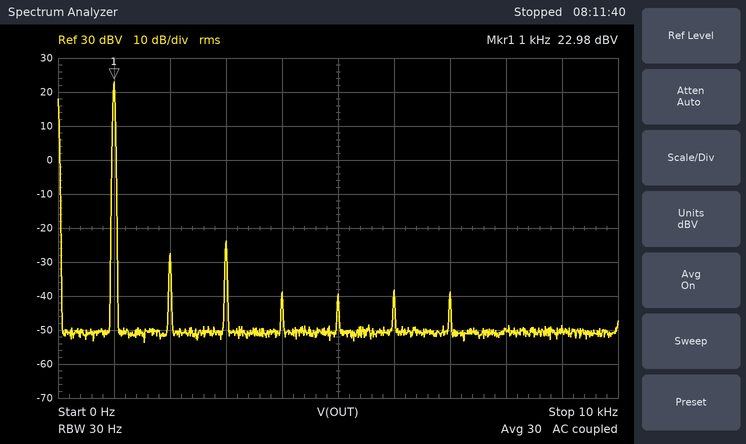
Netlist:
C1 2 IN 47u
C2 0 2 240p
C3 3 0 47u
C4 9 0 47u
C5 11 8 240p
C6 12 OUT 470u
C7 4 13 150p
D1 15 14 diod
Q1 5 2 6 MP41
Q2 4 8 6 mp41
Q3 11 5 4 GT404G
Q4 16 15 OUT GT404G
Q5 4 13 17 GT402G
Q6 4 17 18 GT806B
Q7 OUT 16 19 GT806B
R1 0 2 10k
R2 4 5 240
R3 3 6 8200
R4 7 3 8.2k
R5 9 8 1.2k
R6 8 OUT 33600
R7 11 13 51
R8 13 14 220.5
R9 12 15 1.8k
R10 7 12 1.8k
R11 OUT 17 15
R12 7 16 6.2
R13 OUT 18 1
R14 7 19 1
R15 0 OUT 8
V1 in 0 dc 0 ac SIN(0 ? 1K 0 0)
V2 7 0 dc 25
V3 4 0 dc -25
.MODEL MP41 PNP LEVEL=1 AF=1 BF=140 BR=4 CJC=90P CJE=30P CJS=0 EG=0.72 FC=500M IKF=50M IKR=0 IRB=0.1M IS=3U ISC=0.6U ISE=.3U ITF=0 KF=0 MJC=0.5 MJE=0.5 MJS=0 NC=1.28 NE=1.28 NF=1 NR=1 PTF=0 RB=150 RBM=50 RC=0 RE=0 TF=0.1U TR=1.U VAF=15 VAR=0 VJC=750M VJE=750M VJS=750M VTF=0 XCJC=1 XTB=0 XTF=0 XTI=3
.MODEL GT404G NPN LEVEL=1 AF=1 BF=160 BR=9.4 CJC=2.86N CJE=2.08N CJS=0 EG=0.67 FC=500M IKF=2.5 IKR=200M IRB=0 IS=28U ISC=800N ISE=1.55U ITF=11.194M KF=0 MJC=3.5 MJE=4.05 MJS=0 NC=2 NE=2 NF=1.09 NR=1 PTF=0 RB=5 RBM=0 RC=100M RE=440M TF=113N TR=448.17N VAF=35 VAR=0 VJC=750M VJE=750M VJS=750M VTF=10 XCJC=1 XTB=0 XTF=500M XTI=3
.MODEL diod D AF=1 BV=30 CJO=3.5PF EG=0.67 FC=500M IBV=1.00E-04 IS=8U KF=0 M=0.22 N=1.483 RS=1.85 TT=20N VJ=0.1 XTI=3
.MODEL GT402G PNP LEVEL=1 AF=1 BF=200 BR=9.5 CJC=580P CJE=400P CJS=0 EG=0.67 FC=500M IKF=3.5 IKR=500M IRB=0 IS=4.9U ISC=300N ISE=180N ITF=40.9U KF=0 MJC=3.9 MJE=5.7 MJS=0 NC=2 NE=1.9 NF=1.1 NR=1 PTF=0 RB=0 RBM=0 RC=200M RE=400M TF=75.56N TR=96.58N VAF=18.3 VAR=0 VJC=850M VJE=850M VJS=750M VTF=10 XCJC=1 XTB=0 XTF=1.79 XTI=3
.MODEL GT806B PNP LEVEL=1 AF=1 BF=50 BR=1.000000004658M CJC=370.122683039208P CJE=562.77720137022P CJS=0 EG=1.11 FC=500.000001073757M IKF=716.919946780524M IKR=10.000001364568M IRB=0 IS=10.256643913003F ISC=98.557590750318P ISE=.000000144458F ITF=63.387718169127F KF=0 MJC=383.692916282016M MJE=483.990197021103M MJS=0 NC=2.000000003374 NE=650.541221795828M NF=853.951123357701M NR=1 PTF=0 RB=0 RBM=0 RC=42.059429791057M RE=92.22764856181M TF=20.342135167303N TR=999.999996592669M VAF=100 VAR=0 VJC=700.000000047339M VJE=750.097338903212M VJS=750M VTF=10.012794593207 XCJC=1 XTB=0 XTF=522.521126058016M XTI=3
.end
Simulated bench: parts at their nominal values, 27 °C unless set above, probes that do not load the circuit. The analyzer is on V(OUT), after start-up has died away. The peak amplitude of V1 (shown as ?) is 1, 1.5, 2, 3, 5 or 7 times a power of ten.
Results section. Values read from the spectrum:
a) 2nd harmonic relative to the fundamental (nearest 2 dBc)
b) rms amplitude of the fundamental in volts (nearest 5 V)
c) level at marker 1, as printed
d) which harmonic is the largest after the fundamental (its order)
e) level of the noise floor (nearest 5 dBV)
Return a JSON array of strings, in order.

["-50 dBc", "15 V", "22.98 dBV", "3", "-50 dBV"]
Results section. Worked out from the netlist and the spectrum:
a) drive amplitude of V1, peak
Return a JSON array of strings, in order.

["700 mV"]
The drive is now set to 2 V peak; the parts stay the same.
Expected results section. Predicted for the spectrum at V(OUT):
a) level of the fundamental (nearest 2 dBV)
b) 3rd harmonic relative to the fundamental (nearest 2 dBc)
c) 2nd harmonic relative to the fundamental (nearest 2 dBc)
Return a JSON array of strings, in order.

["26 dBV", "-12 dBc", "-34 dBc"]
